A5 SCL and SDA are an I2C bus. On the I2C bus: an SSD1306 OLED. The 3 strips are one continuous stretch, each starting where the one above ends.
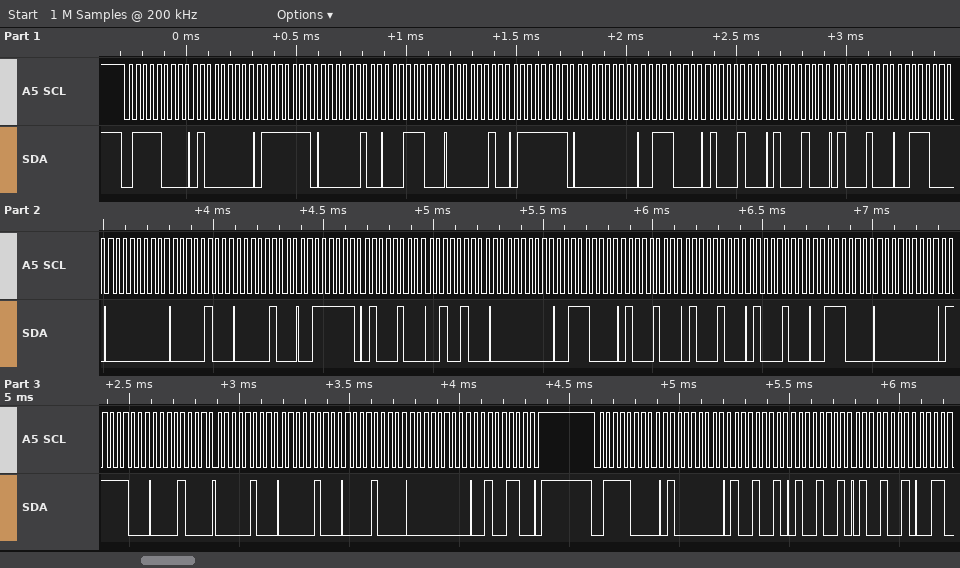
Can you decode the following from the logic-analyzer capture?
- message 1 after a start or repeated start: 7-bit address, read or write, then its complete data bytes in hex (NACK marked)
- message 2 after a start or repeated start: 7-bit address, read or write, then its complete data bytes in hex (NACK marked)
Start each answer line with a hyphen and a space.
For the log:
- 0x3C write: 40 7F 02 1C 02 7F 00 38 44 44 44 38 00 04 04 3F 44 24 00 38 44 44 44 38 00 7C 08 04 04 08 00 26
- 0x3C write: 40 49 49 49
